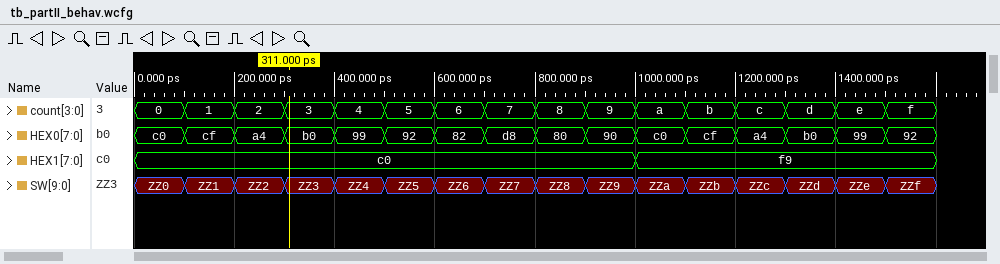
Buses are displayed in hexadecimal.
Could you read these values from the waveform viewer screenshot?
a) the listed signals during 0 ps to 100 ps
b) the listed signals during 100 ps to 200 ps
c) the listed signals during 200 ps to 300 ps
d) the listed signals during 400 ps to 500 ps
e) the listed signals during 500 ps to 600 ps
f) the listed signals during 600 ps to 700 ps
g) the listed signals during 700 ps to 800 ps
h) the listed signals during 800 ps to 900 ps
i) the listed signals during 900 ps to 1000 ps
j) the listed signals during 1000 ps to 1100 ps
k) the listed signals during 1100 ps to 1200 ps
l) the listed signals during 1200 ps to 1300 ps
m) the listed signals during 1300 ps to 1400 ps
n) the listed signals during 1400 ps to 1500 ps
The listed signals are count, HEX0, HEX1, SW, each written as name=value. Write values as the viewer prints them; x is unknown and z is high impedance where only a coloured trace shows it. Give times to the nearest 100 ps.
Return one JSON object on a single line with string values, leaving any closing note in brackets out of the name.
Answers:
{"the listed signals during 0 ps to 100 ps": "count=0, HEX0=c0, HEX1=c0, SW=ZZ0", "the listed signals during 100 ps to 200 ps": "count=1, HEX0=cf, HEX1=c0, SW=ZZ1", "the listed signals during 200 ps to 300 ps": "count=2, HEX0=a4, HEX1=c0, SW=ZZ2", "the listed signals during 400 ps to 500 ps": "count=4, HEX0=99, HEX1=c0, SW=ZZ4", "the listed signals during 500 ps to 600 ps": "count=5, HEX0=92, HEX1=c0, SW=ZZ5", "the listed signals during 600 ps to 700 ps": "count=6, HEX0=82, HEX1=c0, SW=ZZ6", "the listed signals during 700 ps to 800 ps": "count=7, HEX0=d8, HEX1=c0, SW=ZZ7", "the listed signals during 800 ps to 900 ps": "count=8, HEX0=80, HEX1=c0, SW=ZZ8", "the listed signals during 900 ps to 1000 ps": "count=9, HEX0=90, HEX1=c0, SW=ZZ9", "the listed signals during 1000 ps to 1100 ps": "count=a, HEX0=c0, HEX1=f9, SW=ZZa", "the listed signals during 1100 ps to 1200 ps": "count=b, HEX0=cf, HEX1=f9, SW=ZZb", "the listed signals during 1200 ps to 1300 ps": "count=c, HEX0=a4, HEX1=f9, SW=ZZc", "the listed signals during 1300 ps to 1400 ps": "count=d, HEX0=b0, HEX1=f9, SW=ZZd", "the listed signals during 1400 ps to 1500 ps": "count=e, HEX0=99, HEX1=f9, SW=ZZe"}
